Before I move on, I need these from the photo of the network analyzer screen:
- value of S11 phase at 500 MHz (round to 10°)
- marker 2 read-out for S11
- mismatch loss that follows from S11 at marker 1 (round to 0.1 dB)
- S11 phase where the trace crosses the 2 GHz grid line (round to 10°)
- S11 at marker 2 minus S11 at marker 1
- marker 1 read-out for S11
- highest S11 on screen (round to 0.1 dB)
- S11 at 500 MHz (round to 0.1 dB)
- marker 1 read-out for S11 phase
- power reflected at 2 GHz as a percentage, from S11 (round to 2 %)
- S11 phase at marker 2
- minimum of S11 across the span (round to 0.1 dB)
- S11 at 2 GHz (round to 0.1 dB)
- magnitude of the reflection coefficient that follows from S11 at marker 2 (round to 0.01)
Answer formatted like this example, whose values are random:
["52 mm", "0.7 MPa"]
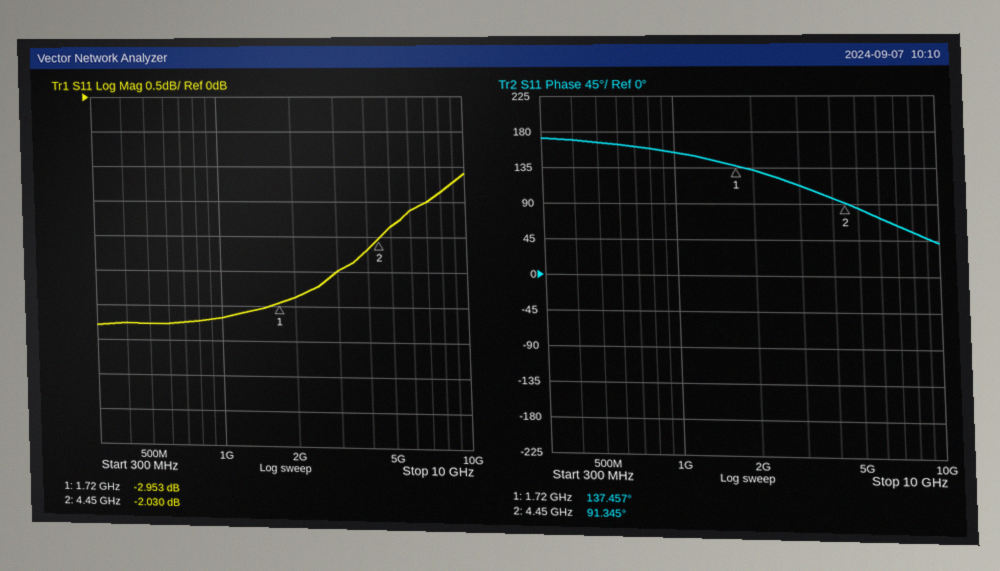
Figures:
["170°", "-2.030 dB", "3.1 dB", "130°", "0.923 dB", "-2.953 dB", "-1.1 dB", "-3.3 dB", "137.457°", "52 %", "91.345°", "-3.3 dB", "-2.9 dB", "0.79"]
